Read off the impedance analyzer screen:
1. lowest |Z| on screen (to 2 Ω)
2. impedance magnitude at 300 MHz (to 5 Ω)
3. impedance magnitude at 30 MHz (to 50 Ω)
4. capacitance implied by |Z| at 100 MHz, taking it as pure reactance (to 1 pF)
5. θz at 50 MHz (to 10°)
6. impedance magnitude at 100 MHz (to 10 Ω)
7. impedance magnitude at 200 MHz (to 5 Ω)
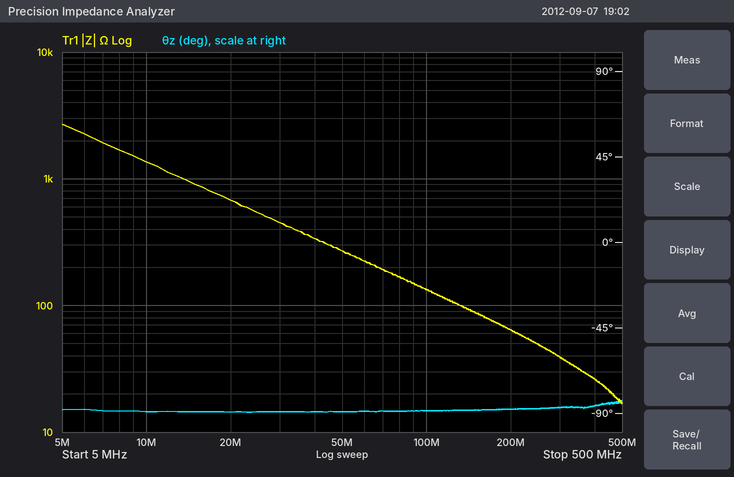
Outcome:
16 Ω
40 Ω
450 Ω
12 pF
-90°
130 Ω
65 Ω
